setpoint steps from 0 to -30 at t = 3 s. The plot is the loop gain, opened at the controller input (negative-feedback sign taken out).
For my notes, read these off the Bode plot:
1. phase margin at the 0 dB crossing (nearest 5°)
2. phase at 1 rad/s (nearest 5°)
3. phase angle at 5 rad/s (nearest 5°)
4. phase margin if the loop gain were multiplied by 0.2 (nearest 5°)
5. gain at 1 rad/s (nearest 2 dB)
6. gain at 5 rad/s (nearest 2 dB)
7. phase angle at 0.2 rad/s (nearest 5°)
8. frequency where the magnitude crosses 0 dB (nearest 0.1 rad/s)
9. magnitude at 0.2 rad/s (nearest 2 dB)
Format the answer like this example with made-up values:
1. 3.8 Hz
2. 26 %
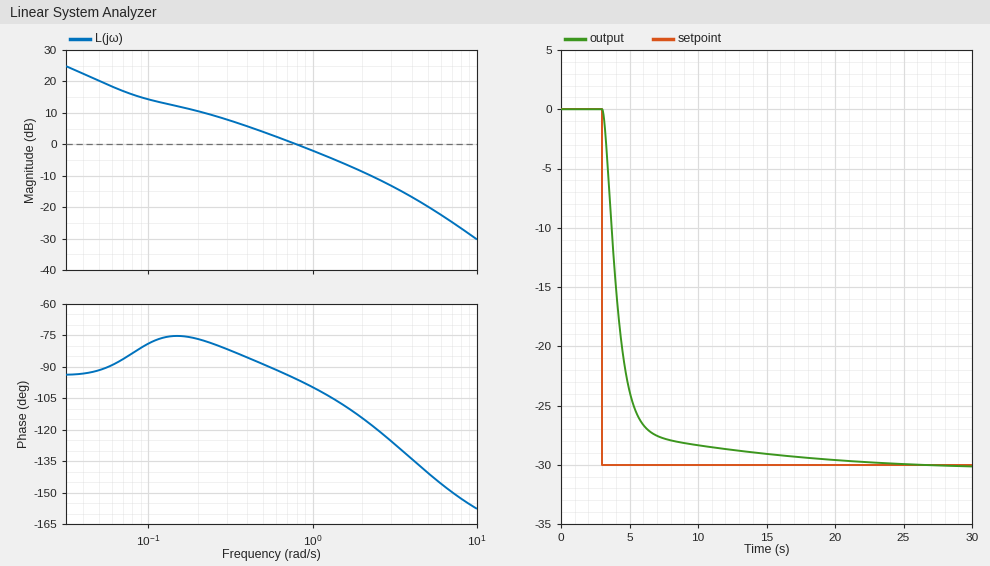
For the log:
1. 85°
2. -100°
3. -140°
4. 100°
5. -2 dB
6. -20 dB
7. -75°
8. 0.8 rad/s
9. 10 dB
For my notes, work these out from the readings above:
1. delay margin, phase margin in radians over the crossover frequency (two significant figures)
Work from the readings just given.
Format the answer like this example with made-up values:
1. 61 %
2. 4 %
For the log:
1. 1.9 s
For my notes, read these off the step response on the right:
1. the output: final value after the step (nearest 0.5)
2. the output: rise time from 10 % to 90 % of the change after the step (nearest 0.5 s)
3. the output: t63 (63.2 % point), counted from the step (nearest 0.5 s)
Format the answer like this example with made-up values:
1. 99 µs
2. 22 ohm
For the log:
1. -30.0
2. 3.0 s
3. 1.5 s
